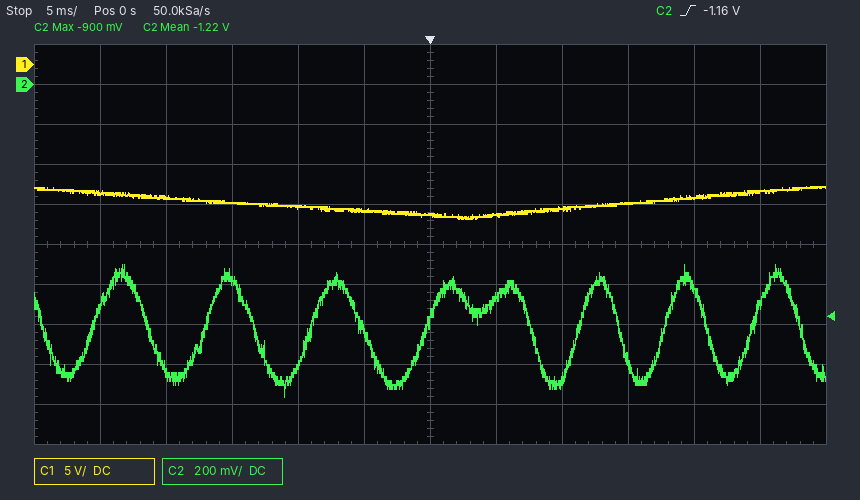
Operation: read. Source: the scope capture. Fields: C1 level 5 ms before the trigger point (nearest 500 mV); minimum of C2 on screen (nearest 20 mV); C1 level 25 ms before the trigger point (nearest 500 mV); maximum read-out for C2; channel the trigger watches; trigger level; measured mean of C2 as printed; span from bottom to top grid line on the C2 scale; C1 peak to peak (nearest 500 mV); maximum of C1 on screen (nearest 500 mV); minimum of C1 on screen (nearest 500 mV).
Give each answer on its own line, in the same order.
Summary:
-18.0 V
-1.56 V
-16.0 V
-900 mV
C2
-1.16 V
-1.22 V
2 V
4.0 V
-15.0 V
-19.0 V
